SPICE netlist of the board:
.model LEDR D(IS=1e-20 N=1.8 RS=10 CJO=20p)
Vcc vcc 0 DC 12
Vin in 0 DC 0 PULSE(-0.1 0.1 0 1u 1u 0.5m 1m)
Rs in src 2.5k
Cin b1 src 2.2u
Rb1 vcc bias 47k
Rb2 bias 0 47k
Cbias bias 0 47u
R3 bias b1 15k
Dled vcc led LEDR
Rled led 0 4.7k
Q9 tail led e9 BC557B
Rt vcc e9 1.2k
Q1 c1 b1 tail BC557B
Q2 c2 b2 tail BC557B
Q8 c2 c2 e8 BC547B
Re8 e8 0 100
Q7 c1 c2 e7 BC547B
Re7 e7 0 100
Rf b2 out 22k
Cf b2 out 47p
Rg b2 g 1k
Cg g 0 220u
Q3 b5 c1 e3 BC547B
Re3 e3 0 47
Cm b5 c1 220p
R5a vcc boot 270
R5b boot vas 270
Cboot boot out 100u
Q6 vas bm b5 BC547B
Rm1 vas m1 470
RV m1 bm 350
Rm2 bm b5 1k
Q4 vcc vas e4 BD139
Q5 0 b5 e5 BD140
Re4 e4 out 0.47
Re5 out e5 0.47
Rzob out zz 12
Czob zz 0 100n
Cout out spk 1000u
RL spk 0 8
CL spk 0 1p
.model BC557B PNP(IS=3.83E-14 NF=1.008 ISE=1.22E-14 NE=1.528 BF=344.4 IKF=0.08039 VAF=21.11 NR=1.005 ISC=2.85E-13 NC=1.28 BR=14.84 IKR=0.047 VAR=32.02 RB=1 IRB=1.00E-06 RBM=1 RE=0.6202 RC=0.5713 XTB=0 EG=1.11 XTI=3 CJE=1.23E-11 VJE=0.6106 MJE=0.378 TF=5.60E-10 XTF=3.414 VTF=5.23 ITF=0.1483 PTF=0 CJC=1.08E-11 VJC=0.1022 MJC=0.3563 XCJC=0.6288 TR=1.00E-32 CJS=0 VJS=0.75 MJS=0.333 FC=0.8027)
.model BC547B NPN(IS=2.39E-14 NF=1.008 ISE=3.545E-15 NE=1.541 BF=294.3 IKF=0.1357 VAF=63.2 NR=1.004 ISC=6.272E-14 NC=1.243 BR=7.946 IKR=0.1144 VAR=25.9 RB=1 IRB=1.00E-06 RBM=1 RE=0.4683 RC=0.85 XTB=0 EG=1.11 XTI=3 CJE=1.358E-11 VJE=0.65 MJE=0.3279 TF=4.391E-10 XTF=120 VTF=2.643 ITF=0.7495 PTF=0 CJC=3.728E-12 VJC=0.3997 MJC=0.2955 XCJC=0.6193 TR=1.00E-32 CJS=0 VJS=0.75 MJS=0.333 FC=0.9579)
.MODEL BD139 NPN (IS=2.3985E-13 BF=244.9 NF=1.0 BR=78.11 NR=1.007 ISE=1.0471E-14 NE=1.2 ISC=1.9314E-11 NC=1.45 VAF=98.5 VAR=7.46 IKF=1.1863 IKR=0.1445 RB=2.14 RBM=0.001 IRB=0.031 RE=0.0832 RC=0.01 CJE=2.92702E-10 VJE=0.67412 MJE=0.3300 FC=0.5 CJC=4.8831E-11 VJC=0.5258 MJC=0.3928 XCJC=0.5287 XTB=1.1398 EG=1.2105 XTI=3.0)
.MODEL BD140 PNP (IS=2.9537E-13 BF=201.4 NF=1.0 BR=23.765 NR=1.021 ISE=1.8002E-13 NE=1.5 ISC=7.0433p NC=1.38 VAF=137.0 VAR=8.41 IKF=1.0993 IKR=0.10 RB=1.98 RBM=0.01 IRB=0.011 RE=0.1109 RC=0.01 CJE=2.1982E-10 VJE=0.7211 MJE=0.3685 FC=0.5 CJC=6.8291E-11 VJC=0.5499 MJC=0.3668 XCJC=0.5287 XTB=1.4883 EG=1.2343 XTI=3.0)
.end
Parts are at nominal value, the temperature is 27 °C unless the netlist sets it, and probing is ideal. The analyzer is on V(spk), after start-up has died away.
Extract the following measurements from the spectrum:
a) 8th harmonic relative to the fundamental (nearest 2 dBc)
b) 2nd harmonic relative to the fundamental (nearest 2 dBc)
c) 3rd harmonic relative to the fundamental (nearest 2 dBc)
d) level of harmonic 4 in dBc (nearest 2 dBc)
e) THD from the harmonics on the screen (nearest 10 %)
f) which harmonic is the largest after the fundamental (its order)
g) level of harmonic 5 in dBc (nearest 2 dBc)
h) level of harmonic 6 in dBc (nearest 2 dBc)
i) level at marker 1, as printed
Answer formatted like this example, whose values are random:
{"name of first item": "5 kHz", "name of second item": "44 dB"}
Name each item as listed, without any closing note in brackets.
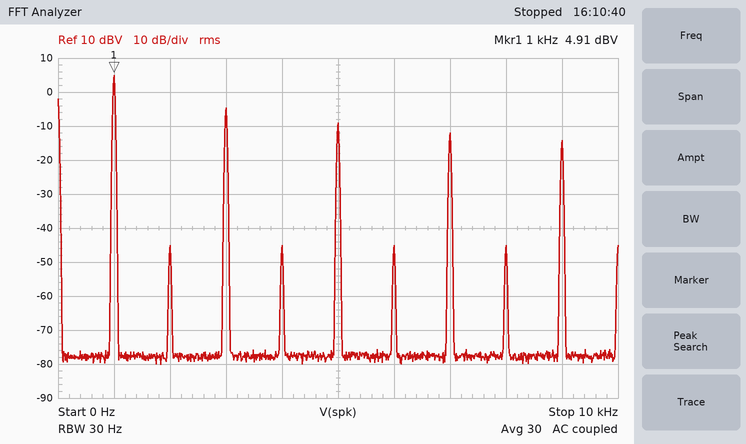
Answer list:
{"8th harmonic relative to the fundamental": "-50 dBc", "2nd harmonic relative to the fundamental": "-50 dBc", "3rd harmonic relative to the fundamental": "-10 dBc", "level of harmonic 4 in dBc": "-50 dBc", "THD from the harmonics on the screen": "40 %", "which harmonic is the largest after the fundamental": "3", "level of harmonic 5 in dBc": "-14 dBc", "level of harmonic 6 in dBc": "-50 dBc", "level at marker 1, as printed": "4.91 dBV"}
